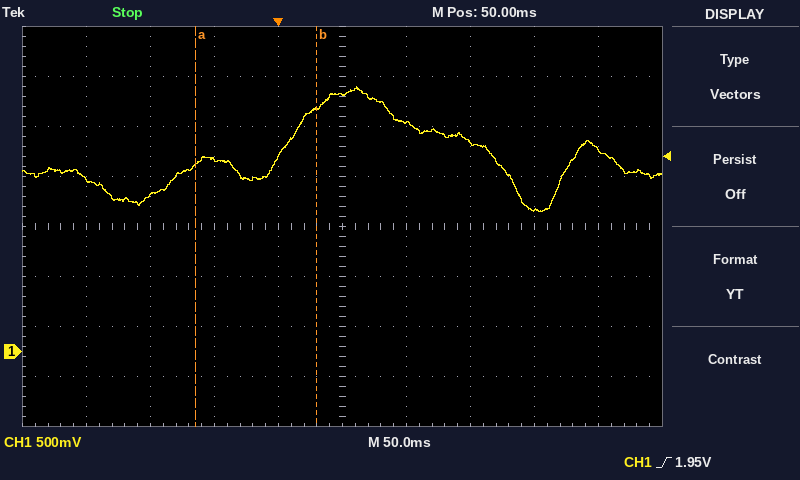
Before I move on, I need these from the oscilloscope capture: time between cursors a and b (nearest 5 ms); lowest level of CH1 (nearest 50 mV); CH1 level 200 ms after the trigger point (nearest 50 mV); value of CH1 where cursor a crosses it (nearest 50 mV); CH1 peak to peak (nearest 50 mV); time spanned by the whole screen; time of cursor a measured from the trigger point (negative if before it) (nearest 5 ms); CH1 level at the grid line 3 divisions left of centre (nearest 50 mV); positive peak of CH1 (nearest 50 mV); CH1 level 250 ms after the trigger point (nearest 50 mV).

95 ms
1.40 V
1.40 V
1.85 V
1.25 V
500 ms
-65 ms
1.55 V
2.65 V
2.00 V
